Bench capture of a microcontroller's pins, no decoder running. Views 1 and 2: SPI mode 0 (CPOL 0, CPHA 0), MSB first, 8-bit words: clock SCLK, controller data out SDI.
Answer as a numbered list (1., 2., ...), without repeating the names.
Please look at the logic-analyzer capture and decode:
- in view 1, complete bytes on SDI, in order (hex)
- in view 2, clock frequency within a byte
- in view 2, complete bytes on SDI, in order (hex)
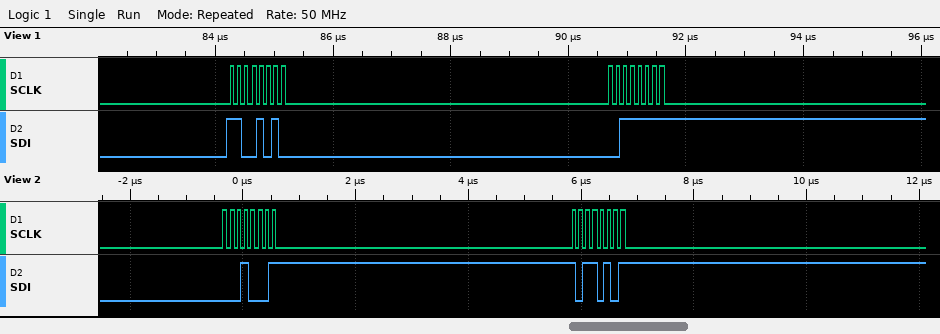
1. 0xCA 0x3F
2. 8 MHz
3. 11 B5
